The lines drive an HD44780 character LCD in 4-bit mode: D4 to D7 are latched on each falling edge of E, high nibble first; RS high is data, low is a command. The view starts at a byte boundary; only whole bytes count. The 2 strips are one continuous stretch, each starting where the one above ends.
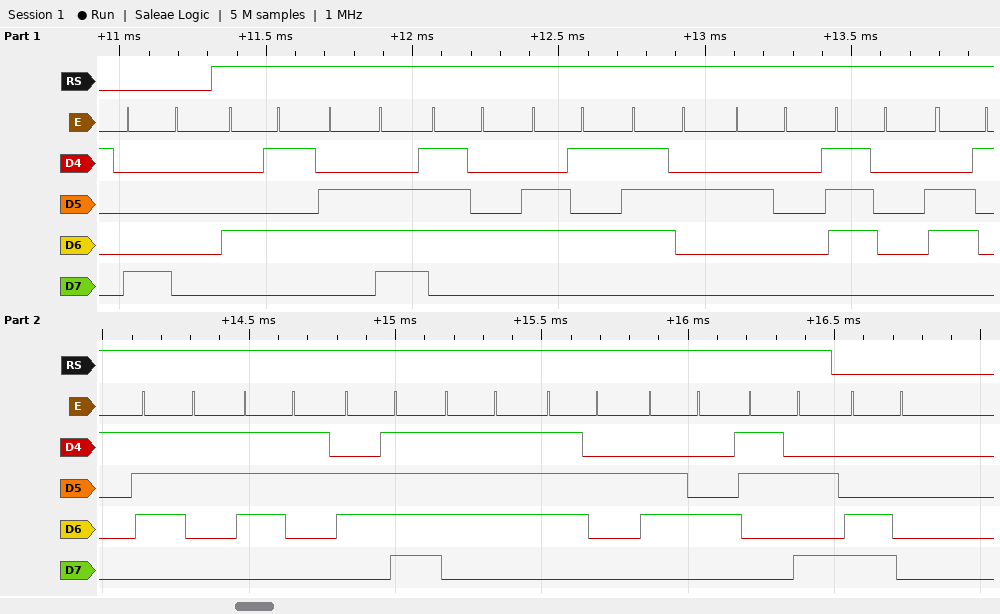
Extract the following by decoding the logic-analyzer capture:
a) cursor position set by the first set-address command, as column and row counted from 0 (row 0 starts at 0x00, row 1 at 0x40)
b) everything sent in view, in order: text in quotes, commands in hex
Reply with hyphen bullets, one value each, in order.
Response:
- column 0, row 0
- 0x80 "Enter passowrd:" 0xC0
